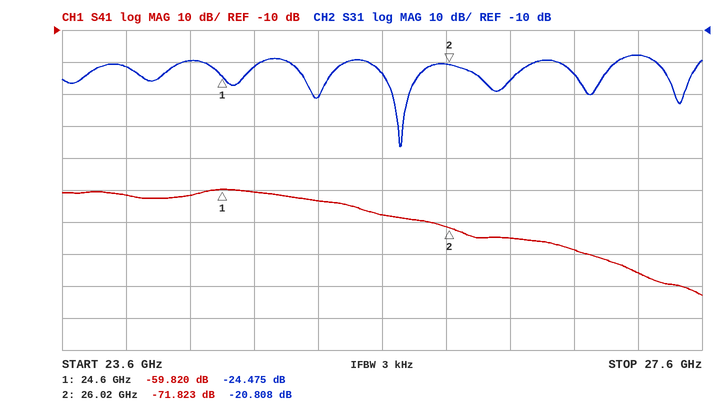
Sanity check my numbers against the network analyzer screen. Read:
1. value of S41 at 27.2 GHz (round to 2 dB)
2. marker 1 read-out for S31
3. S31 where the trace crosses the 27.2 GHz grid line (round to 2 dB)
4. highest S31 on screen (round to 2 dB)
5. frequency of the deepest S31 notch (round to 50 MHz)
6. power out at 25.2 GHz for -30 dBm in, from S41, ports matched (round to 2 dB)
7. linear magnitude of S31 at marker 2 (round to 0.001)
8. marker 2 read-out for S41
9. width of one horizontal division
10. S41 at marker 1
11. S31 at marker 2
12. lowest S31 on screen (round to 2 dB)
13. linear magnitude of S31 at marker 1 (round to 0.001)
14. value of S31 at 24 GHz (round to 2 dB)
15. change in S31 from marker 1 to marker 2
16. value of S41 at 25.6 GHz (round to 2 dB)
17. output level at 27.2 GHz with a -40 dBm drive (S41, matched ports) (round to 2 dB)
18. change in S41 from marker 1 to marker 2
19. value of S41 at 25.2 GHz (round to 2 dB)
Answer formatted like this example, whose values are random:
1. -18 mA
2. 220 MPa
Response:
1. -86 dB
2. -24.475 dB
3. -18 dB
4. -18 dB
5. 25.70 GHz
6. -94 dBm
7. 0.091
8. -71.823 dB
9. 400 MHz
10. -59.820 dB
11. -20.808 dB
12. -46 dB
13. 0.060
14. -22 dB
15. 3.667 dB
16. -68 dB
17. -126 dBm
18. -12.003 dB
19. -64 dB
